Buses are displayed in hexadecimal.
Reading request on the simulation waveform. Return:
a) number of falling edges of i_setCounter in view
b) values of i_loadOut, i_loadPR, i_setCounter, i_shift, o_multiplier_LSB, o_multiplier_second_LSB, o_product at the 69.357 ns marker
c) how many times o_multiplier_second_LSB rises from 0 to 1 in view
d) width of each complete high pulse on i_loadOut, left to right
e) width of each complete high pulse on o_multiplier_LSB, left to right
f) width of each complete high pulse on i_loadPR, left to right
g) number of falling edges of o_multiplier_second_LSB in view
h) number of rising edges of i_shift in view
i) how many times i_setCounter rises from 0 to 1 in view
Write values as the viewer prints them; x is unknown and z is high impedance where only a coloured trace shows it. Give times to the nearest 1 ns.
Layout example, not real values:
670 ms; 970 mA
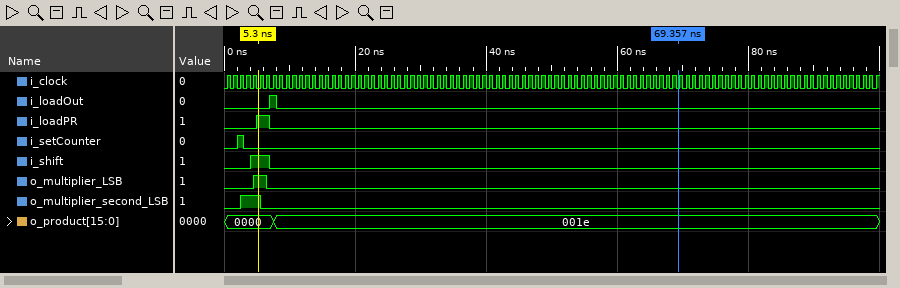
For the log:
1; i_loadOut=0, i_loadPR=0, i_setCounter=0, i_shift=0, o_multiplier_LSB=0, o_multiplier_second_LSB=0, o_product=001e; 1; 1 ns; 2 ns; 2 ns; 1; 1; 1
